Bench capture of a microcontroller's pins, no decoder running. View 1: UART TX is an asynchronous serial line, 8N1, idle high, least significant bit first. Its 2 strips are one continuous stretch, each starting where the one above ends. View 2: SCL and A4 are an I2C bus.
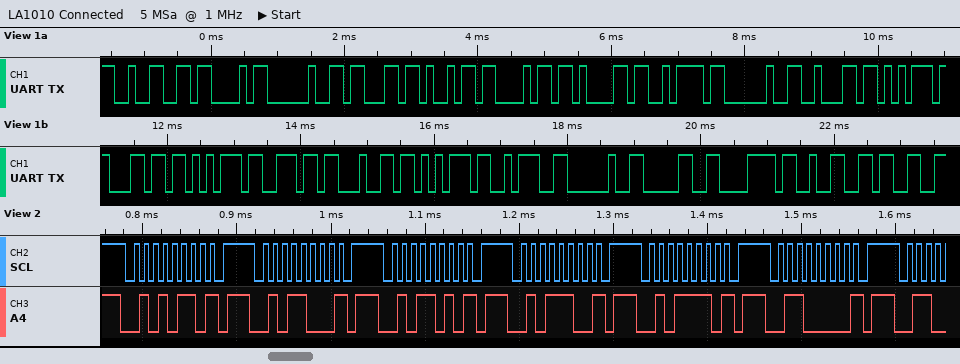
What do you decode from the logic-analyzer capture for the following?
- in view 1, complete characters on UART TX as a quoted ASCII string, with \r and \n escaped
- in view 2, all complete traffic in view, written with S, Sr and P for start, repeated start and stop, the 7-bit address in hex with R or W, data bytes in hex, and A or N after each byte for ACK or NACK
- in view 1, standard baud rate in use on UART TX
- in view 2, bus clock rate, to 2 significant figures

"2C cihaz bulundu: 0x23"
S 2BW N P S 2CW N P S 2DW N P S 2EW N P S 2FW N P S 30W N P
9600 baud
100 kHz
